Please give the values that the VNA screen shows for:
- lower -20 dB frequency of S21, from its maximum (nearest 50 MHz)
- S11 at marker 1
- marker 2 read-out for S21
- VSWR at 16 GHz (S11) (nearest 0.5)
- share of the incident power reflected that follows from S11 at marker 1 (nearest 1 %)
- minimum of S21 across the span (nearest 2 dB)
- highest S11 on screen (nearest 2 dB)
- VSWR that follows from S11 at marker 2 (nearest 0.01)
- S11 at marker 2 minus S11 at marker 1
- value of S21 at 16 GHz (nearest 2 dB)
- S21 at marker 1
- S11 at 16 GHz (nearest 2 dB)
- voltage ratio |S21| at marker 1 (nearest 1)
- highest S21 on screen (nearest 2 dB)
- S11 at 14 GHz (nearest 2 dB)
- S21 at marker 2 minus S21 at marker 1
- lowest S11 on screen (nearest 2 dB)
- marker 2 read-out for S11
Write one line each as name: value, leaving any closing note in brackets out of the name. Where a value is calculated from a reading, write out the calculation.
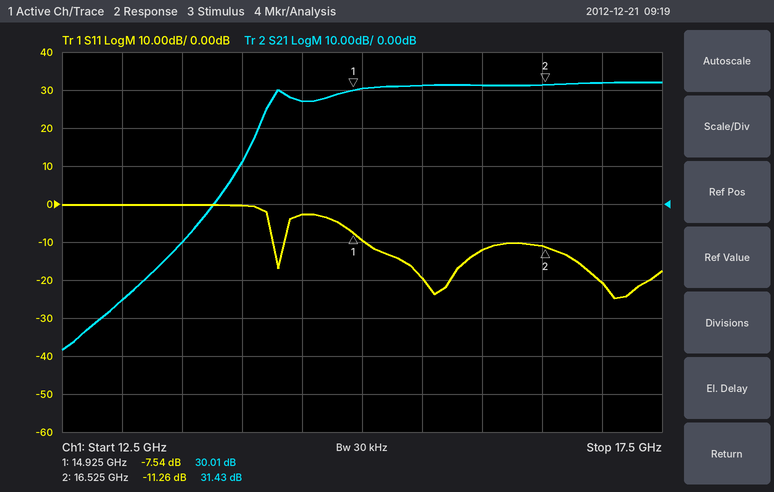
lower -20 dB frequency of S21, from its maximum: 14.00 GHz
S11 at marker 1: -7.54 dB
marker 2 read-out for S21: 31.43 dB
VSWR at 16 GHz (S11): |Γ| = 10^(-12/20) = 0.2512; VSWR = (1 + 0.2512)/(1 − 0.2512) ≈ 1.67, so 1.5 to the nearest 0.5
share of the incident power reflected that follows from S11 at marker 1: 10^(-7.54/10) ≈ 18 %
minimum of S21 across the span: -38 dB
highest S11 on screen: 0 dB
VSWR that follows from S11 at marker 2: (1 + 0.2735)/(1 − 0.2735) ≈ 1.75
S11 at marker 2 minus S11 at marker 1: -11.26 − (-7.54) = -3.72 dB
value of S21 at 16 GHz: 32 dB
S21 at marker 1: 30.01 dB
S11 at 16 GHz: -12 dB
voltage ratio |S21| at marker 1: 10^(30.01/20) ≈ 32
highest S21 on screen: 32 dB
S11 at 14 GHz: 0 dB
S21 at marker 2 minus S21 at marker 1: 31.43 − (30.01) = 1.42 dB
lowest S11 on screen: -24 dB
marker 2 read-out for S11: -11.26 dB
